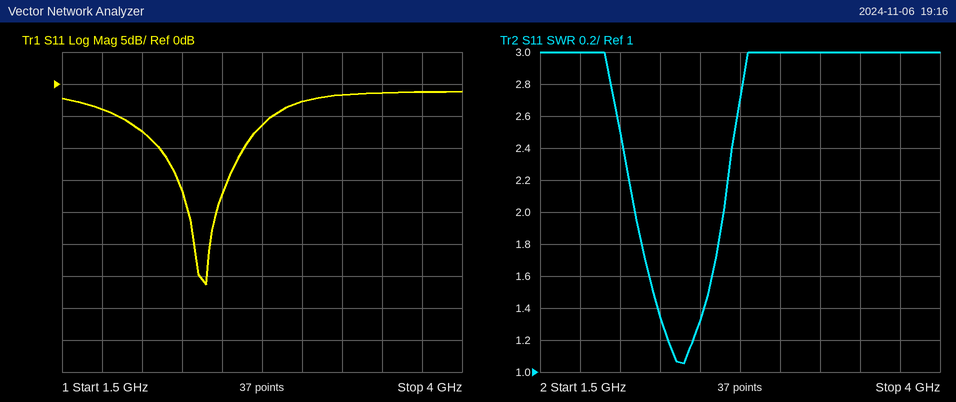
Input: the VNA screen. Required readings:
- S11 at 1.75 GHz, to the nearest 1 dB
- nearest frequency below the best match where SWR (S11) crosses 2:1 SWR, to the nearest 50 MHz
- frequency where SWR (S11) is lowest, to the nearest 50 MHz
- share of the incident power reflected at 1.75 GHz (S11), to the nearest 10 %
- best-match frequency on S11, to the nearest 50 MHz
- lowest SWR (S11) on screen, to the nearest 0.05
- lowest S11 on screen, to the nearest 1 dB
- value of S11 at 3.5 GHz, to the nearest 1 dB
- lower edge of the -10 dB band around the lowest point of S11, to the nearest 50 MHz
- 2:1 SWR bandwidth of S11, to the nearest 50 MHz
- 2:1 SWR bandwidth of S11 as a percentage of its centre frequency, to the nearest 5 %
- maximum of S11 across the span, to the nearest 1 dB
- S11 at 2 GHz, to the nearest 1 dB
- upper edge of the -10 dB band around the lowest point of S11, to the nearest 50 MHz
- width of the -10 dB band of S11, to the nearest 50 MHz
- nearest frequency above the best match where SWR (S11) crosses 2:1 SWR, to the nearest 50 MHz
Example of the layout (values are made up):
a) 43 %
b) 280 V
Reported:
a) -4 dB
b) 2.10 GHz
c) 2.40 GHz
d) 40 %
e) 2.40 GHz
f) 1.05
g) -31 dB
h) -1 dB
i) 2.10 GHz
j) 550 MHz
k) 25 %
l) -1 dB
m) -7 dB
n) 2.65 GHz
o) 550 MHz
p) 2.65 GHz
